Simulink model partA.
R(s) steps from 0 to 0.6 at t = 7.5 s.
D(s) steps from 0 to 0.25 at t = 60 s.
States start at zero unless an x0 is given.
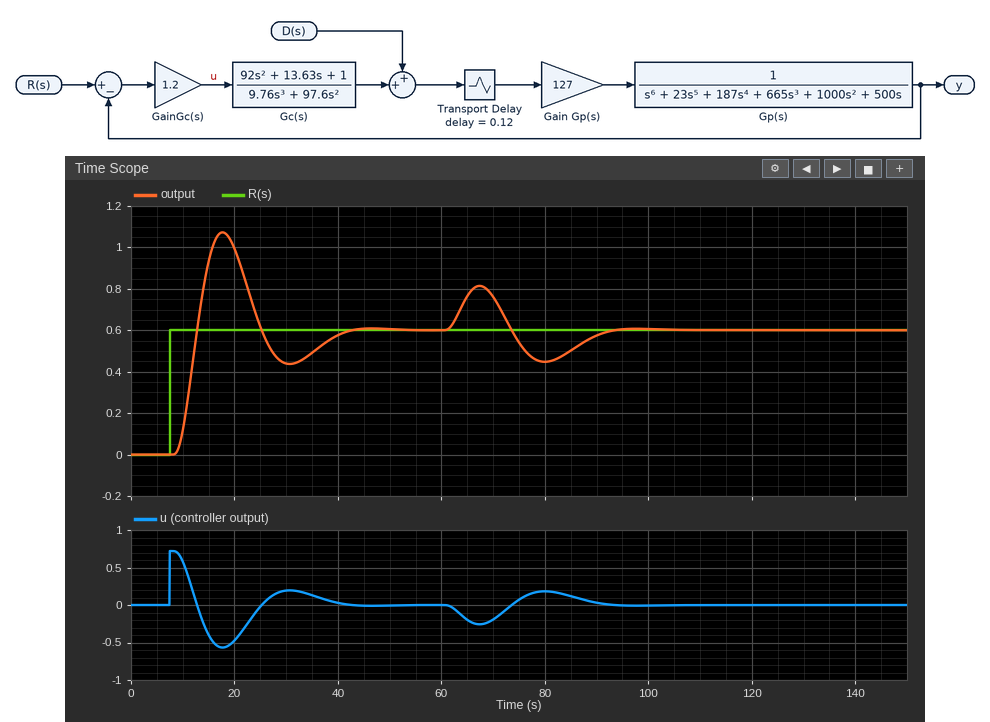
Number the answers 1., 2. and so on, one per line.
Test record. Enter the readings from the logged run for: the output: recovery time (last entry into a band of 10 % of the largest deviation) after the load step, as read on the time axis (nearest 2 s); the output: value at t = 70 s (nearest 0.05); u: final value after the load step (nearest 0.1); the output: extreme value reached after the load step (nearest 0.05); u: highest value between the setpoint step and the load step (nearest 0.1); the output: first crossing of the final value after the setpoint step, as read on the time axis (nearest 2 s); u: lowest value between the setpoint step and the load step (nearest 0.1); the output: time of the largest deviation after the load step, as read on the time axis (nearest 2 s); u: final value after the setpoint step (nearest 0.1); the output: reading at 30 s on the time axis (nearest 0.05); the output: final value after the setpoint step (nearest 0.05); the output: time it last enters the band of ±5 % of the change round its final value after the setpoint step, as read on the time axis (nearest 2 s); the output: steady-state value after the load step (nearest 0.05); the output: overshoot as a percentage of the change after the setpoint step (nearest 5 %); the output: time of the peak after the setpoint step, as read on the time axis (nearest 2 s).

1. 90 s
2. 0.75
3. 0.0
4. 0.80
5. 0.7
6. 12 s
7. -0.6
8. 68 s
9. 0.0
10. 0.45
11. 0.60
12. 40 s
13. 0.60
14. 80 %
15. 18 s
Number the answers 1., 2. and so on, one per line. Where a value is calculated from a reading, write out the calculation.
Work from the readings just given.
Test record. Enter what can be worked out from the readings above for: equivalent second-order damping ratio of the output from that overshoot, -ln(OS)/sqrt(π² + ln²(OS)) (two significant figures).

1. ln(0.8) = -0.223; 0.223 / sqrt(9.870 + 0.050) = 0.071
